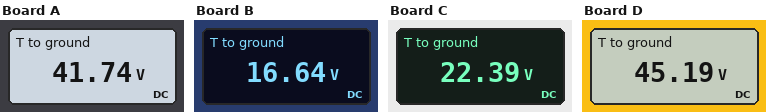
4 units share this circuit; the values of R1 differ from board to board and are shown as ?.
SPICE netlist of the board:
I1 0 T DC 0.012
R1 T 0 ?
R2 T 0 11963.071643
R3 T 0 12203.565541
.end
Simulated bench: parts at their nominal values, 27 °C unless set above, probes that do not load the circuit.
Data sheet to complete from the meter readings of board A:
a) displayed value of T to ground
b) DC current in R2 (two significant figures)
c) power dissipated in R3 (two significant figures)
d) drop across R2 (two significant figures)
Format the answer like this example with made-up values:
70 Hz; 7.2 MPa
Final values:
41.74 V; 3.5 mA; 140 mW; 42 V
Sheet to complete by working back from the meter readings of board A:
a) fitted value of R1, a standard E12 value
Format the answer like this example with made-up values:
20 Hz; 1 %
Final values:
8.2 kΩ
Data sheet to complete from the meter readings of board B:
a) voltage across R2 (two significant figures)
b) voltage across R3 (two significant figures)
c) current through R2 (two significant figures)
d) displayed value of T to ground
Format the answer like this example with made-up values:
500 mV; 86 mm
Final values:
17 V; 17 V; 1.4 mA; 16.64 V
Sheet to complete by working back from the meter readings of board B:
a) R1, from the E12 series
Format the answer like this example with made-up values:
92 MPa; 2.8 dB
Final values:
1.8 kΩ
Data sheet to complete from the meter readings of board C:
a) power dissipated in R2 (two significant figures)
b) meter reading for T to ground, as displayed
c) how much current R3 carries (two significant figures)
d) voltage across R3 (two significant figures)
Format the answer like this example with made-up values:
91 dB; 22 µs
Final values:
42 mW; 22.39 V; 1.8 mA; 22 V
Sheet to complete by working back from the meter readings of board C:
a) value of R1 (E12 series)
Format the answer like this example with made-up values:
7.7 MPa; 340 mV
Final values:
2.7 kΩ
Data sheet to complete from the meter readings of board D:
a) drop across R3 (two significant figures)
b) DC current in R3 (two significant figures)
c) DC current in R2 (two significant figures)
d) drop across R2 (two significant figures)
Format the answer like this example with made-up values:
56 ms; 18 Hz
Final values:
45 V; 3.7 mA; 3.8 mA; 45 V
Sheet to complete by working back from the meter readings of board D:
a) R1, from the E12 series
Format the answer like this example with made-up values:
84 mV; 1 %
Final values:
10 kΩ
